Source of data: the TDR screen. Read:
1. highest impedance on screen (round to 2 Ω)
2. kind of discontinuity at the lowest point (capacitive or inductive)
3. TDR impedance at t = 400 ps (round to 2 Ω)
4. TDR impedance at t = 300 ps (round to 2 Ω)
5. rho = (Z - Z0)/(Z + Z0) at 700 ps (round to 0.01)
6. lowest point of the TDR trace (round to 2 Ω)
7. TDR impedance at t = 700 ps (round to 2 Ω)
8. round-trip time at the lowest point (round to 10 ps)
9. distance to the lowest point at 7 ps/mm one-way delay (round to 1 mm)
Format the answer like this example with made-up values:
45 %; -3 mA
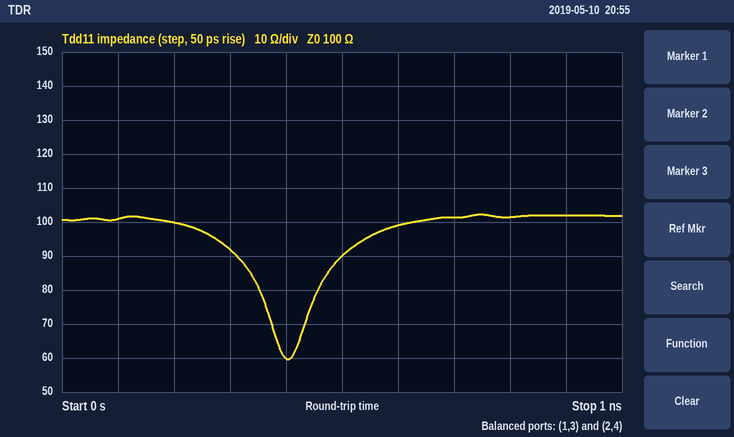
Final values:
102 Ω; capacitive; 60 Ω; 92 Ω; +0.01; 60 Ω; 102 Ω; 400 ps; 29 mm
